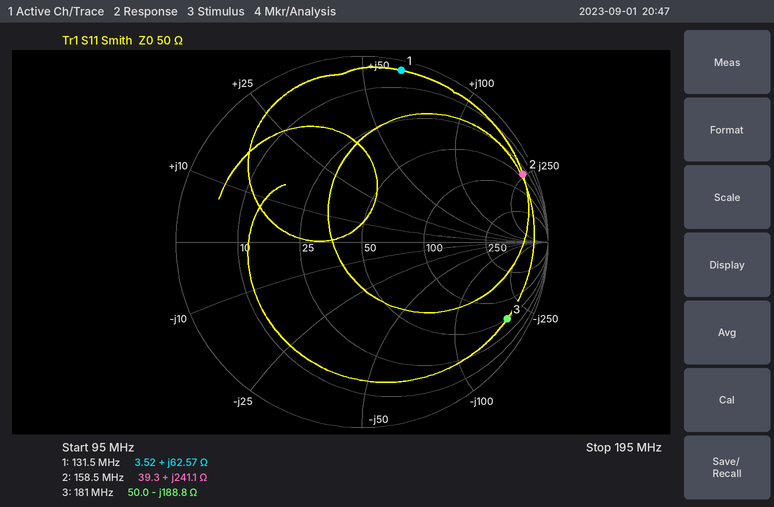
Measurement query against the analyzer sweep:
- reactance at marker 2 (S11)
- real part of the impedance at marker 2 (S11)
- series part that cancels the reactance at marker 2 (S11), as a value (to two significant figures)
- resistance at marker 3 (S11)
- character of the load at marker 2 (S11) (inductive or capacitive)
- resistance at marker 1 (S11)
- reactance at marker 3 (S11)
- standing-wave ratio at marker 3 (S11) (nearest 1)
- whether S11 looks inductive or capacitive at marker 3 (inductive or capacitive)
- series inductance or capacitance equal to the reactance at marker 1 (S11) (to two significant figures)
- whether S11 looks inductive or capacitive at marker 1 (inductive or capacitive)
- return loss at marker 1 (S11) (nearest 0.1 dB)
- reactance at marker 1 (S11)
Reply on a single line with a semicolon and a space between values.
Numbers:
+241.1 Ω; 39.3 Ω; 4.2 pF; 50.0 Ω; inductive; 3.52 Ω; -188.8 Ω; 16; capacitive; 76 nH; inductive; 0.5 dB; +62.57 Ω
